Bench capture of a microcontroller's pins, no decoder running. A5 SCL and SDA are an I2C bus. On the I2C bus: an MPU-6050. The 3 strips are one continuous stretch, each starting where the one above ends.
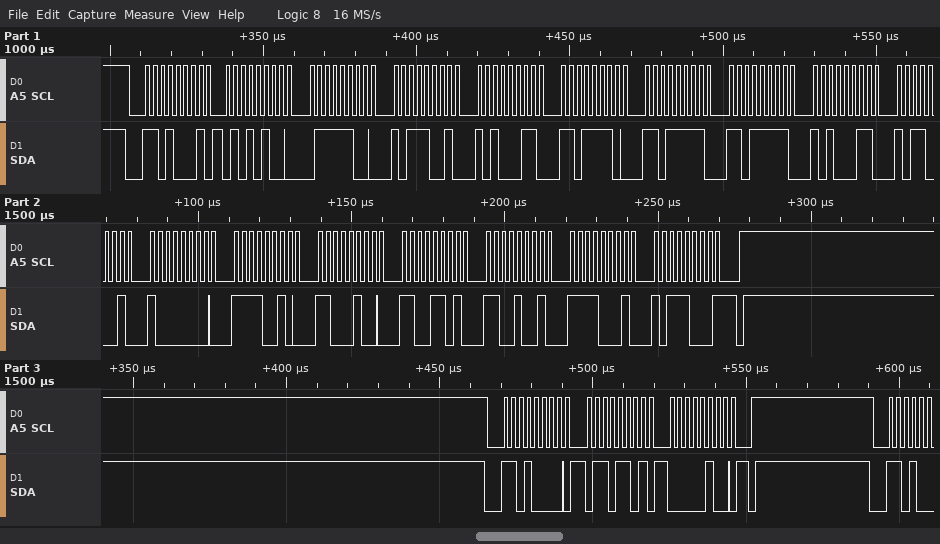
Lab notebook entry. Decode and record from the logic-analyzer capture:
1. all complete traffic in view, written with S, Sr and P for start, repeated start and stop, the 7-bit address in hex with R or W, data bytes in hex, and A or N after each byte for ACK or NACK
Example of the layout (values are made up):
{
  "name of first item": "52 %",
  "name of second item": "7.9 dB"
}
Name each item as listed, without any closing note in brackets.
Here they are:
{
  "all complete traffic in view, written with S, Sr and P for start, repeated start and stop, the 7-bit address in hex with R or W, data bytes in hex, and A or N after each byte for ACK or NACK": "S 68R A 54 A 7C A B9 A A3 A DE A DF A DF A A3 A B1 A 80 A F2 A C4 A CD A C9 A F1 A B8 N P S 68W A 6D A 04 A P"
}
